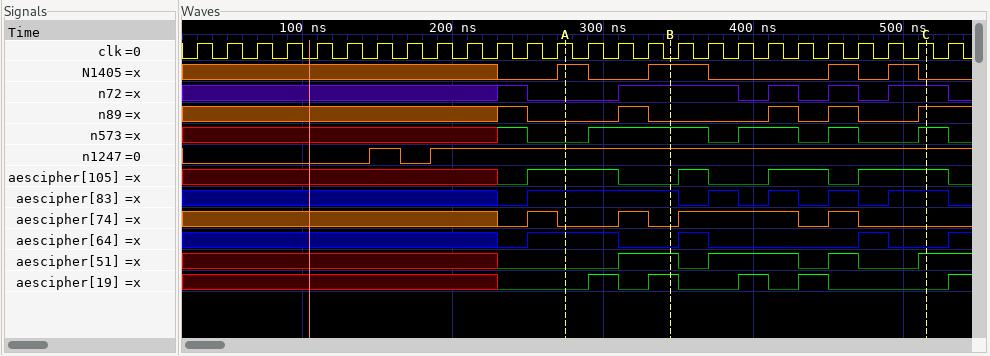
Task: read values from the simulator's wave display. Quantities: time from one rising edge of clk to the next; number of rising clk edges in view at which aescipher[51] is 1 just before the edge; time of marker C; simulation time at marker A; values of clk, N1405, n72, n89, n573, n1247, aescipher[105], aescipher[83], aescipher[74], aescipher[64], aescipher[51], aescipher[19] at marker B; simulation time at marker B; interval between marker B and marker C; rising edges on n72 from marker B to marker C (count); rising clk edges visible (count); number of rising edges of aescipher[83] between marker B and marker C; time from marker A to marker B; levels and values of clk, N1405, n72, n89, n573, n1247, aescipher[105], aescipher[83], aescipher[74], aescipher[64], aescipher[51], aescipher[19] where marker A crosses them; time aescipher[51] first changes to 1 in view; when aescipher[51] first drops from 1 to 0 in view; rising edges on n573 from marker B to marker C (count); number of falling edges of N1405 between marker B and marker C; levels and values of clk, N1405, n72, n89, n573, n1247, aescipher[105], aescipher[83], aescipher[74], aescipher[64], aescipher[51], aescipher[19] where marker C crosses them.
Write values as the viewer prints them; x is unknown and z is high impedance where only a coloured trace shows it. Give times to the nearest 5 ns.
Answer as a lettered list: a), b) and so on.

a) 20 ns
b) 7
c) 515 ns
d) 275 ns
e) clk=0, N1405=1, n72=1, n89=0, n573=1, n1247=1, aescipher[105]=0, aescipher[83]=1, aescipher[74]=0, aescipher[64]=0, aescipher[51]=1, aescipher[19]=1
f) 345 ns
g) 170 ns
h) 3
i) 26
j) 4
k) 70 ns
l) clk=1, N1405=1, n72=0, n89=0, n573=0, n1247=1, aescipher[105]=1, aescipher[83]=1, aescipher[74]=0, aescipher[64]=1, aescipher[51]=0, aescipher[19]=0
m) 310 ns
n) 350 ns
o) 3
p) 3
q) clk=1, N1405=0, n72=1, n89=1, n573=1, n1247=1, aescipher[105]=1, aescipher[83]=1, aescipher[74]=0, aescipher[64]=0, aescipher[51]=1, aescipher[19]=0
